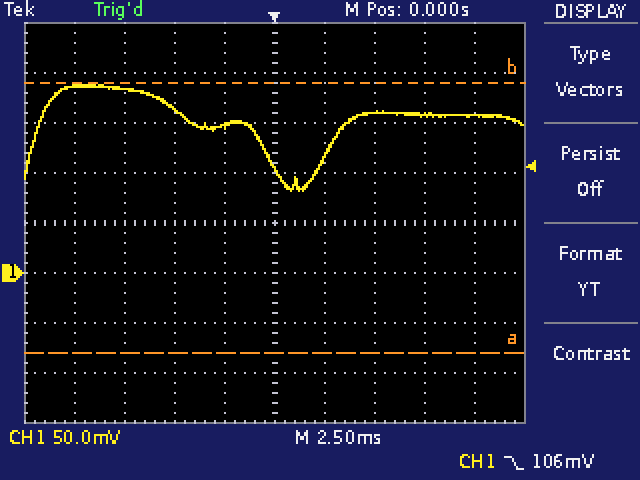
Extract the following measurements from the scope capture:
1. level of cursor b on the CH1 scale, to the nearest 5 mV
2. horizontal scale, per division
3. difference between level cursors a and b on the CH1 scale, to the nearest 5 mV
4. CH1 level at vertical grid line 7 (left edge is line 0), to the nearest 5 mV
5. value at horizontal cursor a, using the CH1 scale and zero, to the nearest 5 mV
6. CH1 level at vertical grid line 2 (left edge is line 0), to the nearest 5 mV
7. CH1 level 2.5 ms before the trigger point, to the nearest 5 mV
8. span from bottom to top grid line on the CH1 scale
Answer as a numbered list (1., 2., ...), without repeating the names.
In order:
1. 190 mV
2. 2.5 ms
3. 270 mV
4. 160 mV
5. -80 mV
6. 185 mV
7. 145 mV
8. 400 mV
